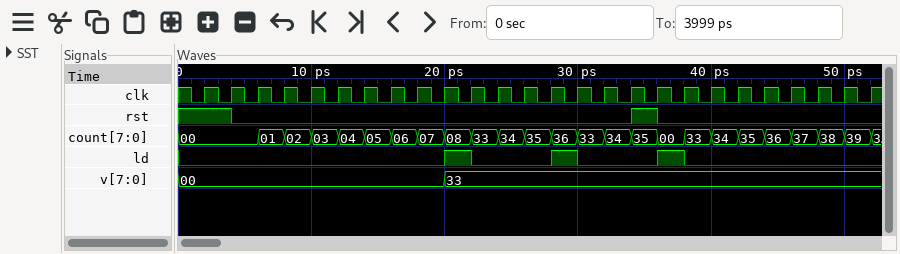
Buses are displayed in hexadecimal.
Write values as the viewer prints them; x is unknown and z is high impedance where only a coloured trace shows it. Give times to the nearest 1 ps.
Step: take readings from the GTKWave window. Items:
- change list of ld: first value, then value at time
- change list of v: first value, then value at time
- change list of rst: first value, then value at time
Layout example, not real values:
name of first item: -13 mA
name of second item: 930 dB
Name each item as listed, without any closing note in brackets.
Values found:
change list of ld: first value, then value at time: 0, 1 at 20 ps, 0 at 22 ps, 1 at 28 ps, 0 at 30 ps, 1 at 36 ps, 0 at 38 ps
change list of v: first value, then value at time: 00, 33 at 20 ps
change list of rst: first value, then value at time: 1, 0 at 4 ps, 1 at 34 ps, 0 at 36 ps
